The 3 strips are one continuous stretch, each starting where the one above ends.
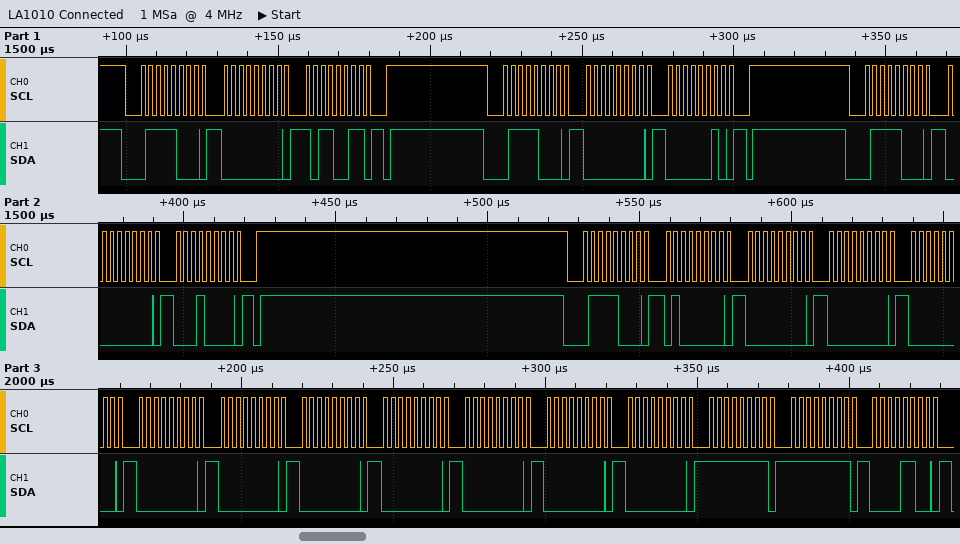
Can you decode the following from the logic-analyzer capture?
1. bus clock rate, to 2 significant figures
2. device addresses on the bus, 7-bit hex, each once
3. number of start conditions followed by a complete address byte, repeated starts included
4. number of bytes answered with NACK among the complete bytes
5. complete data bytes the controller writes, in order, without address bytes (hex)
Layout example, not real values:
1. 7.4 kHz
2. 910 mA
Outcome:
1. 400 kHz
2. 0x3C
3. 4
4. 0
5. 00 B3 00 02 00 10 40 00 00 00 00 00 00 00 00 00 00 FF FF 0C
